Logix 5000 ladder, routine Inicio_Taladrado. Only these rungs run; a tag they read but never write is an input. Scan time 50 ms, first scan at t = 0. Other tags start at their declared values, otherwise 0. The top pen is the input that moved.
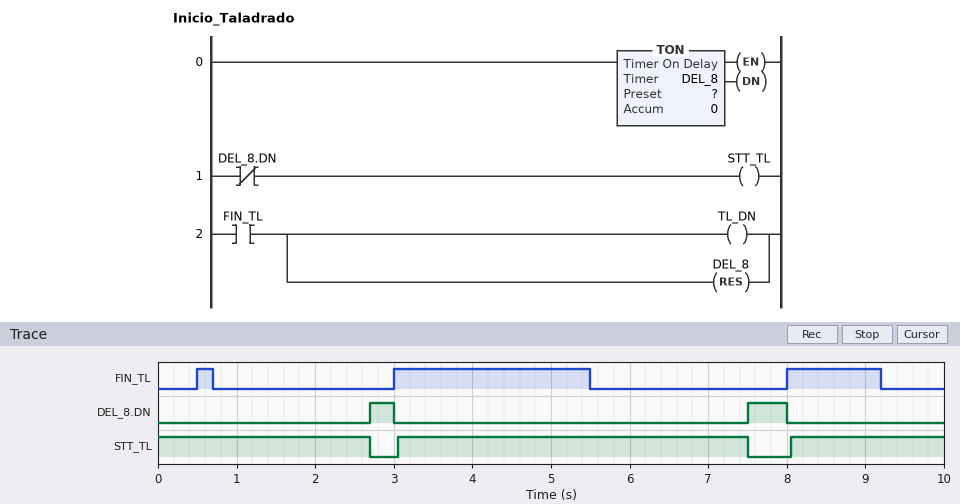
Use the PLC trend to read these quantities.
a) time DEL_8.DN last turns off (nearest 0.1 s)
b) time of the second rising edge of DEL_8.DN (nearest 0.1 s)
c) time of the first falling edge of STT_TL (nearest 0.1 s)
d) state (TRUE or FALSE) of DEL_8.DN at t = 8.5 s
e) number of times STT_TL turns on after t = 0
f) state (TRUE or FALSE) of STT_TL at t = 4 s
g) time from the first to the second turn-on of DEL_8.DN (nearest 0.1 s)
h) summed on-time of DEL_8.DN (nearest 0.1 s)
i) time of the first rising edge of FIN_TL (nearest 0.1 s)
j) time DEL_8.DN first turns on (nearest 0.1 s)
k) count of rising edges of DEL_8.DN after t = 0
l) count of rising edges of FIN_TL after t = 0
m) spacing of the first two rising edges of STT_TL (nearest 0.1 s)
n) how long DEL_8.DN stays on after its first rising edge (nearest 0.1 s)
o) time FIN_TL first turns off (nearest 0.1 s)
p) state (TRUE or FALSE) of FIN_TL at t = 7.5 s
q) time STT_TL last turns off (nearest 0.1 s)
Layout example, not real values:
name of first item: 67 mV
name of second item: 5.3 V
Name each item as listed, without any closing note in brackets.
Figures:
time DEL_8.DN last turns off: 8.0 s
time of the second rising edge of DEL_8.DN: 7.5 s
time of the first falling edge of STT_TL: 2.7 s
state (TRUE or FALSE) of DEL_8.DN at t = 8.5 s: FALSE
number of times STT_TL turns on after t = 0: 2
state (TRUE or FALSE) of STT_TL at t = 4 s: TRUE
time from the first to the second turn-on of DEL_8.DN: 4.8 s
summed on-time of DEL_8.DN: 0.8 s
time of the first rising edge of FIN_TL: 0.5 s
time DEL_8.DN first turns on: 2.7 s
count of rising edges of DEL_8.DN after t = 0: 2
count of rising edges of FIN_TL after t = 0: 3
spacing of the first two rising edges of STT_TL: 5.0 s
how long DEL_8.DN stays on after its first rising edge: 0.3 s
time FIN_TL first turns off: 0.7 s
state (TRUE or FALSE) of FIN_TL at t = 7.5 s: FALSE
time STT_TL last turns off: 7.5 s
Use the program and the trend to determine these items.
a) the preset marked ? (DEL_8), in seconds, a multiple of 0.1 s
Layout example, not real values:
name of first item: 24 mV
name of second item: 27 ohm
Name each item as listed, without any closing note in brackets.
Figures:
the preset marked ? (DEL_8), in seconds, a multiple of 0.1 s: 2.0 s
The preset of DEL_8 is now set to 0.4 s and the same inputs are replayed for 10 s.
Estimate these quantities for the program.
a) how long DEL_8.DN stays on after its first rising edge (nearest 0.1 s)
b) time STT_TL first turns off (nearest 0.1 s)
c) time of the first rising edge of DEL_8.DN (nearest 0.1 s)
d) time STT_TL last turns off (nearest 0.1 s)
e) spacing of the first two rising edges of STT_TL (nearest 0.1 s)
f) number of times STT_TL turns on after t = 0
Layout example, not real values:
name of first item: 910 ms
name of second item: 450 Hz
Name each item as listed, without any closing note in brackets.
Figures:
how long DEL_8.DN stays on after its first rising edge: 0.1 s
time STT_TL first turns off: 0.4 s
time of the first rising edge of DEL_8.DN: 0.4 s
time STT_TL last turns off: 9.6 s
spacing of the first two rising edges of STT_TL: 2.5 s
number of times STT_TL turns on after t = 0: 3
